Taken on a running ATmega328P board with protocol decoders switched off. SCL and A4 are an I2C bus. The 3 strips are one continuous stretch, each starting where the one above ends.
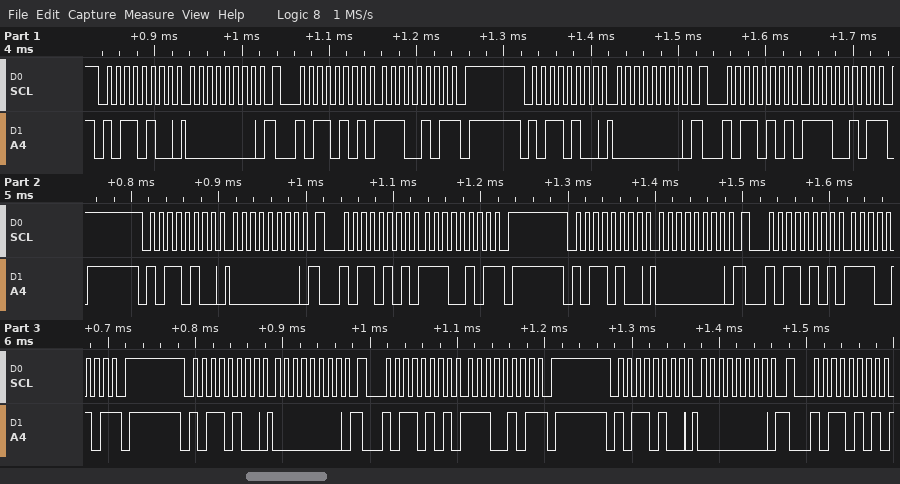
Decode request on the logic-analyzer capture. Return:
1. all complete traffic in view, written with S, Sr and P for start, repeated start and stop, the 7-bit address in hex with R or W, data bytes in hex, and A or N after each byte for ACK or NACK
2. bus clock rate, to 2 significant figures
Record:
S 5AW A 00 A Sr 5AR A E5 N P S 5AW A 00 A Sr 5AR A E5 N P S 5AW A 00 A Sr 5AR A E5 N P S 5AW A 00 A Sr 5AR A E5 N P S 5AW A 00 A Sr 5AR A E5 N P S 5AW A 00 A Sr 5AR A
100 kHz
